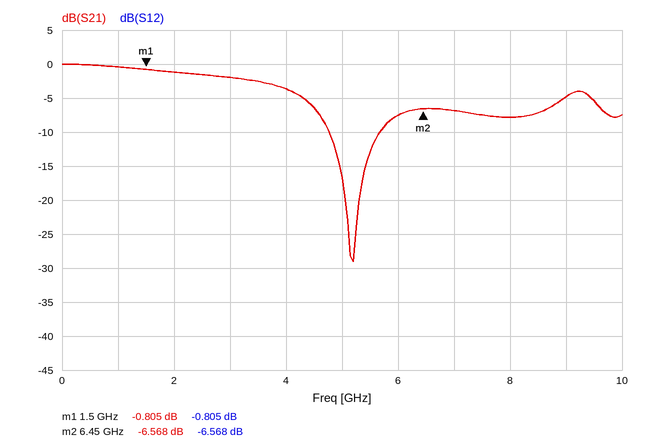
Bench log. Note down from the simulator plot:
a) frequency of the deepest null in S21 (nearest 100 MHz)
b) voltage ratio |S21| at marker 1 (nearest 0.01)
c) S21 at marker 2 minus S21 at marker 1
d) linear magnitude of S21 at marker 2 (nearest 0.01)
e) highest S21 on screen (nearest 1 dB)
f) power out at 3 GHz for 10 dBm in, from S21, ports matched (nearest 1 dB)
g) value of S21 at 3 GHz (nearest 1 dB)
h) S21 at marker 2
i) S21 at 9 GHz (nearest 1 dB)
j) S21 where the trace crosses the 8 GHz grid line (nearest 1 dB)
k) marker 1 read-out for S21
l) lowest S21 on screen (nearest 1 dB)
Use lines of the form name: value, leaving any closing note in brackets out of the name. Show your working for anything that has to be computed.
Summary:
frequency of the deepest null in S21: 5.2 GHz
voltage ratio |S21| at marker 1: 10^(-0.805/20) ≈ 0.91
S21 at marker 2 minus S21 at marker 1: -6.568 − (-0.805) = -5.763 dB
linear magnitude of S21 at marker 2: 10^(-6.568/20) ≈ 0.47
highest S21 on screen: 0 dB
power out at 3 GHz for 10 dBm in, from S21, ports matched: 10 dBm + (-2 dB) = 8 dBm
value of S21 at 3 GHz: -2 dB
S21 at marker 2: -6.568 dB
S21 at 9 GHz: -5 dB
S21 where the trace crosses the 8 GHz grid line: -8 dB
marker 1 read-out for S21: -0.805 dB
lowest S21 on screen: -29 dB
